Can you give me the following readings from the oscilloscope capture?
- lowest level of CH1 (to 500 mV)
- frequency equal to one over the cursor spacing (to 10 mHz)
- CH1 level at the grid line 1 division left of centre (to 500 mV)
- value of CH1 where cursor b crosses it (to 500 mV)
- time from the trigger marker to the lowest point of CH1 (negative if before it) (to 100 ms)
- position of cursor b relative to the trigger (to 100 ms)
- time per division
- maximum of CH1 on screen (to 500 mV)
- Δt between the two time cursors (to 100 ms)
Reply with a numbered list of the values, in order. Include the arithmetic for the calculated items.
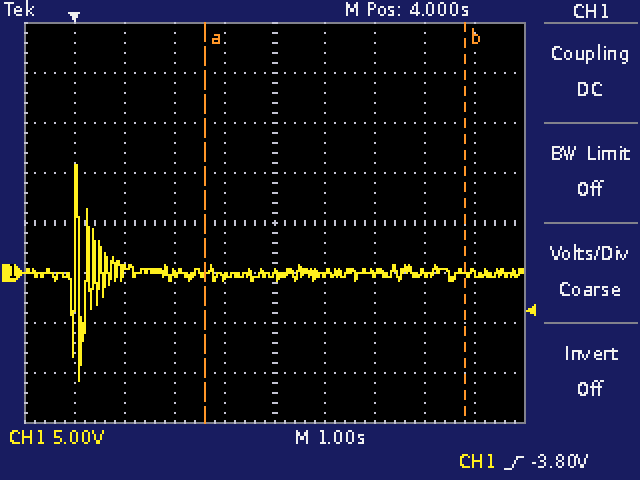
1. -11.0 V
2. 1 / 5.2 s ≈ 190 mHz
3. -500 mV
4. 0.0 V
5. +100 ms
6. +7.8 s
7. 1 s
8. 11.0 V
9. 5.2 s
